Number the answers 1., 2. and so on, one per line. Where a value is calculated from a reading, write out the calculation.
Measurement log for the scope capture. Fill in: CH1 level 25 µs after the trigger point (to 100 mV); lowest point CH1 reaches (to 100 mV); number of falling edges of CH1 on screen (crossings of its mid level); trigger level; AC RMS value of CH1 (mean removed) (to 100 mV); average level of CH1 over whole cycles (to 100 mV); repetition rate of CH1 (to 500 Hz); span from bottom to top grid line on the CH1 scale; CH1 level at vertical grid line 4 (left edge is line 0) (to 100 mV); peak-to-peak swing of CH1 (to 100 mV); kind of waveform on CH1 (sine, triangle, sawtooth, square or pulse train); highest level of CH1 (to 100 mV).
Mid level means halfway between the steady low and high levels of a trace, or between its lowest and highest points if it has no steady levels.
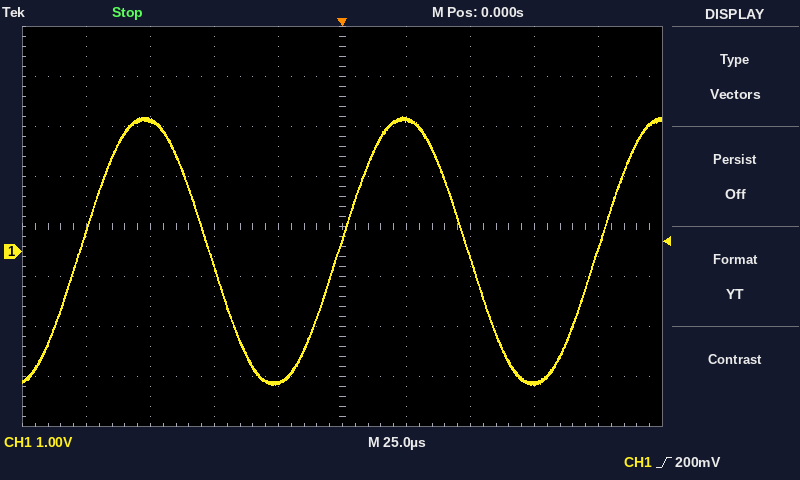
1. 2.6 V
2. -2.7 V
3. 2
4. 200 mV
5. 5.4 V / (2√2) ≈ 1.9 V
6. (2.7 V + (-2.7 V)) / 2 ≈ 0.0 V
7. 10.0 kHz
8. 8 V
9. -2.6 V
10. 2.7 V − (-2.7 V) = 5.4 V
11. sine
12. 2.7 V
